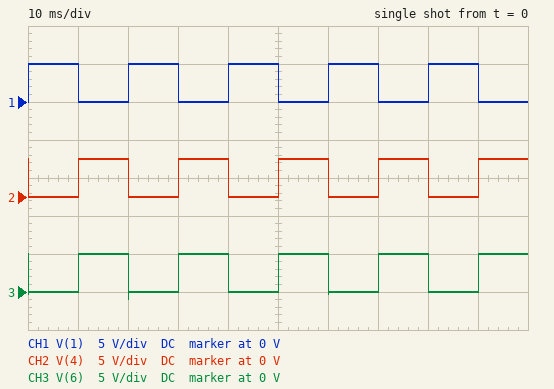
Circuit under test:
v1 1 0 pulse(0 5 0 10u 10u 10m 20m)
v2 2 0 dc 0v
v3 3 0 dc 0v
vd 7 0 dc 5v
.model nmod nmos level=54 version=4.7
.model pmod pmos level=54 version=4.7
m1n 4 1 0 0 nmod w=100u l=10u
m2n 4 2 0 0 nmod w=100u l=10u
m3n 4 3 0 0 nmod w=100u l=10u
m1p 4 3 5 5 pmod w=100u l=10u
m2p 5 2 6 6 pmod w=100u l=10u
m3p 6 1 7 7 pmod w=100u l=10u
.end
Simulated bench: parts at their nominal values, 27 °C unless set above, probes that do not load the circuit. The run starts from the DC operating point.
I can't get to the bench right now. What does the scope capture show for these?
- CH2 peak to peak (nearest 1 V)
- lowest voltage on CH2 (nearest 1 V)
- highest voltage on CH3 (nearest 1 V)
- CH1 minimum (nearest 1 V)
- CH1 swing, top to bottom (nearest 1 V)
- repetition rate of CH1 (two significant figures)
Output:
5 V
0 V
5 V
0 V
5 V
50 Hz
